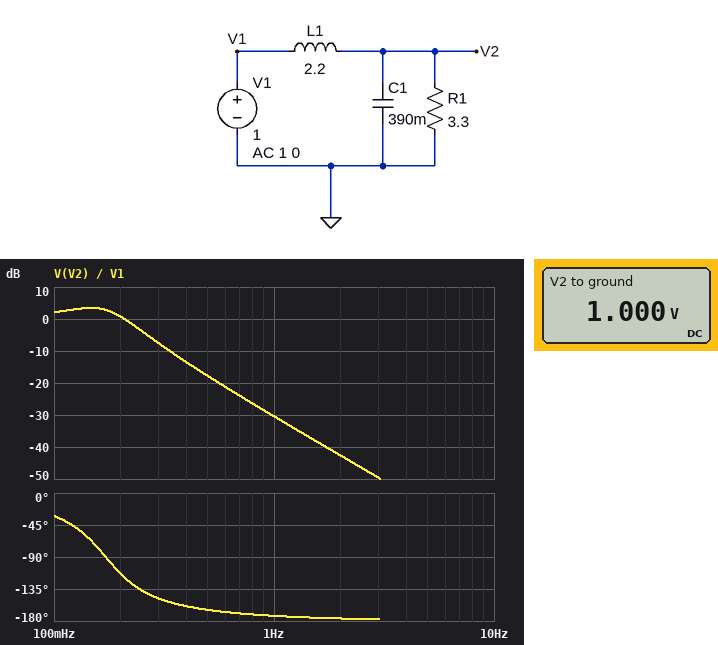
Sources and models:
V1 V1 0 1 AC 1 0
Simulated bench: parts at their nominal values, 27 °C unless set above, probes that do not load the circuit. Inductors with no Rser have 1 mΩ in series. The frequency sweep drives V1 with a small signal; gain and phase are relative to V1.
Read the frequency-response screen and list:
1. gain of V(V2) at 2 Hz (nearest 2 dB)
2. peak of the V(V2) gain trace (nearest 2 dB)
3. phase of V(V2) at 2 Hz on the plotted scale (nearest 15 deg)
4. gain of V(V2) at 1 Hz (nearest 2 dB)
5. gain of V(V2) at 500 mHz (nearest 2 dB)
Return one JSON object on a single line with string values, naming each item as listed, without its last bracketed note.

{"gain of V(V2) at 2 Hz": "-42 dB", "peak of the V(V2) gain trace": "4 dB", "phase of V(V2) at 2 Hz on the plotted scale": "-180 deg", "gain of V(V2) at 1 Hz": "-30 dB", "gain of V(V2) at 500 mHz": "-18 dB"}
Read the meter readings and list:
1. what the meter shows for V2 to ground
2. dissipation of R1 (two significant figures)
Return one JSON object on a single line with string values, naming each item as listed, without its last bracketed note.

{"what the meter shows for V2 to ground": "1.000 V", "dissipation of R1": "300 mW"}
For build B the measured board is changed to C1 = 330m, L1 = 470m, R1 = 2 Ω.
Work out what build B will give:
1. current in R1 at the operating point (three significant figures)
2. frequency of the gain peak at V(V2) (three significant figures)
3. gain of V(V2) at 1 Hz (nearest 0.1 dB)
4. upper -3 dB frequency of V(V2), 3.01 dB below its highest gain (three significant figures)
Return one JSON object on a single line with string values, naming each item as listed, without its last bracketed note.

{"current in R1 at the operating point": "500 mA", "frequency of the gain peak at V(V2)": "366 mHz", "gain of V(V2) at 1 Hz": "-14.5 dB", "upper -3 dB frequency of V(V2), 3.01 dB below its highest gain": "477 mHz"}
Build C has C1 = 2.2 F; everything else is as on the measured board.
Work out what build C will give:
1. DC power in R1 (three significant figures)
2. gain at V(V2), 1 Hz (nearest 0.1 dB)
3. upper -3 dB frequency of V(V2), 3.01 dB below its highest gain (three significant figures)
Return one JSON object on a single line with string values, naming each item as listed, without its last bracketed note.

{"DC power in R1": "303 mW", "gain at V(V2), 1 Hz": "-45.6 dB", "upper -3 dB frequency of V(V2), 3.01 dB below its highest gain": "81.0 mHz"}
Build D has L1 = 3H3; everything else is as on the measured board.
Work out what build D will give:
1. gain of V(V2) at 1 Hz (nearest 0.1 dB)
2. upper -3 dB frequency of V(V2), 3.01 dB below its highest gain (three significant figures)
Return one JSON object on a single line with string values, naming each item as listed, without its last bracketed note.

{"gain of V(V2) at 1 Hz": "-34.0 dB", "upper -3 dB frequency of V(V2), 3.01 dB below its highest gain": "166 mHz"}
